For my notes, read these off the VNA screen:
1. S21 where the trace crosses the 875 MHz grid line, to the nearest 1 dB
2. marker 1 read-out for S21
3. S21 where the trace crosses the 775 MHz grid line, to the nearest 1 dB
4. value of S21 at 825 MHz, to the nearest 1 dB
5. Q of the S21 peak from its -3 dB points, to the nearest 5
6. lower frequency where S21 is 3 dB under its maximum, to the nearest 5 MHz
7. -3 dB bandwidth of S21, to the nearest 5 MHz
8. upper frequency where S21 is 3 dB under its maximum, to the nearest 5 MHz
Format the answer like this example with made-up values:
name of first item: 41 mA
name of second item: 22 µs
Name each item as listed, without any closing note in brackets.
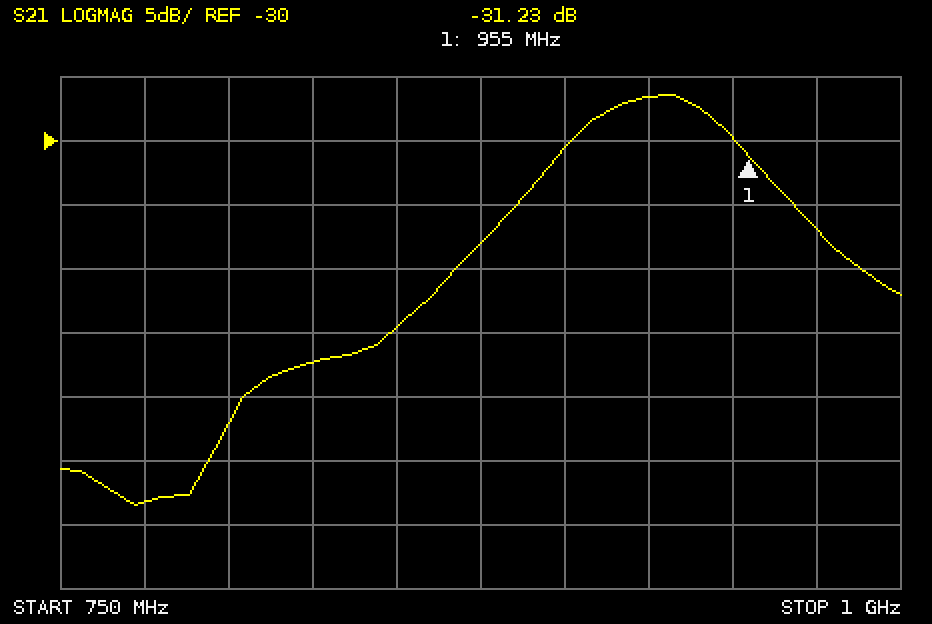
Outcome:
S21 where the trace crosses the 875 MHz grid line, to the nearest 1 dB: -38 dB
marker 1 read-out for S21: -31.23 dB
S21 where the trace crosses the 775 MHz grid line, to the nearest 1 dB: -58 dB
value of S21 at 825 MHz, to the nearest 1 dB: -47 dB
Q of the S21 peak from its -3 dB points, to the nearest 5: 20
lower frequency where S21 is 3 dB under its maximum, to the nearest 5 MHz: 905 MHz
-3 dB bandwidth of S21, to the nearest 5 MHz: 45 MHz
upper frequency where S21 is 3 dB under its maximum, to the nearest 5 MHz: 950 MHz
